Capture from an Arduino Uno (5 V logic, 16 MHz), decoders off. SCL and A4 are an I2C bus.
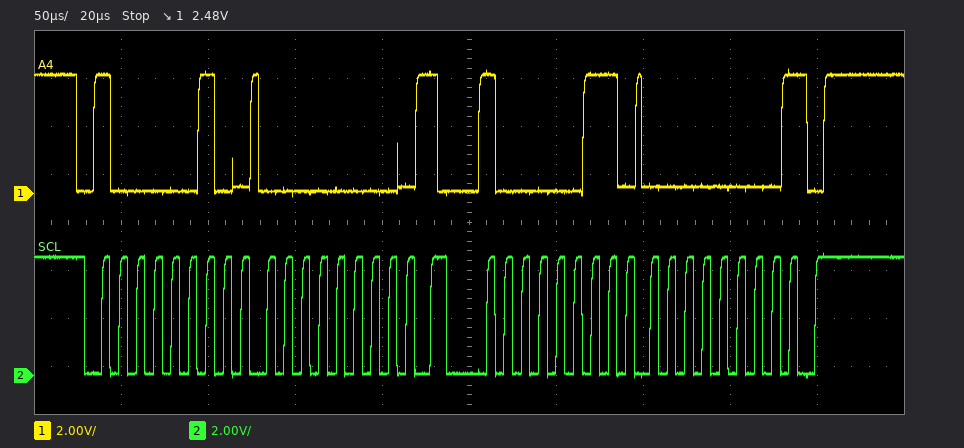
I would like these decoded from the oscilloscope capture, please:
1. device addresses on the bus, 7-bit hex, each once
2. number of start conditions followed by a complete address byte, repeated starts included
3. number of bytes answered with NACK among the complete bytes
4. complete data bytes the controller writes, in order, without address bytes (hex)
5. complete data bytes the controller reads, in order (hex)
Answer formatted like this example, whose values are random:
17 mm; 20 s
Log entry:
0x41; 2; 1; 00; 00
